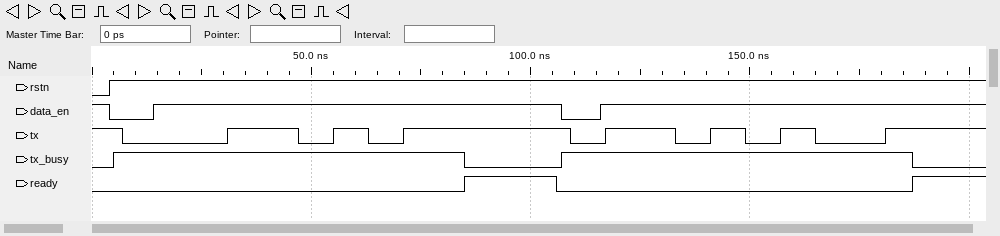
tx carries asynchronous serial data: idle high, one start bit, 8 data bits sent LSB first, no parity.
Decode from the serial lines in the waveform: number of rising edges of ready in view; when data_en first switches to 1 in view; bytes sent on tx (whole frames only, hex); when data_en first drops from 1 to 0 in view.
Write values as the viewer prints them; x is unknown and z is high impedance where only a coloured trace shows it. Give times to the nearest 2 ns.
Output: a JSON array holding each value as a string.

["2", "14 ns", "AC, 2B", "4 ns"]
